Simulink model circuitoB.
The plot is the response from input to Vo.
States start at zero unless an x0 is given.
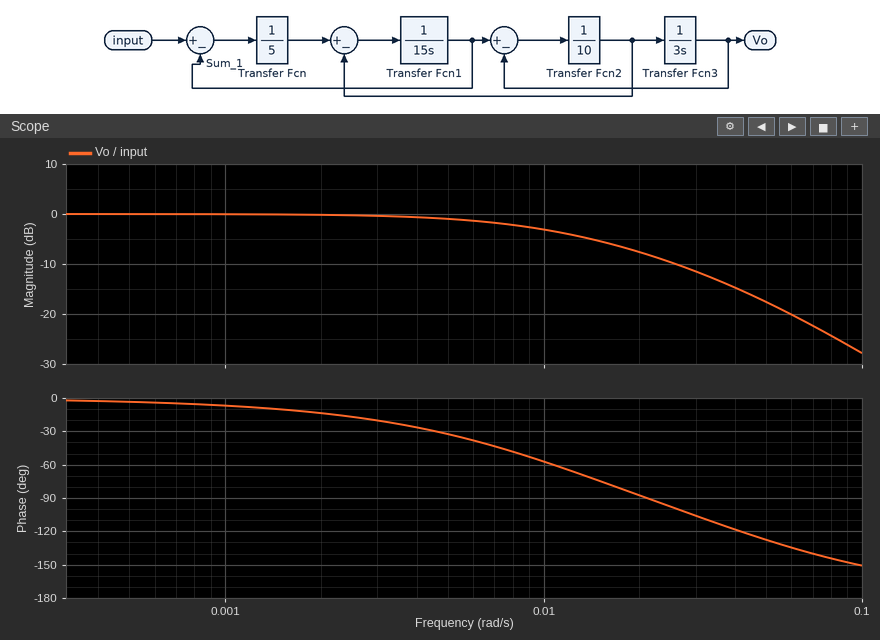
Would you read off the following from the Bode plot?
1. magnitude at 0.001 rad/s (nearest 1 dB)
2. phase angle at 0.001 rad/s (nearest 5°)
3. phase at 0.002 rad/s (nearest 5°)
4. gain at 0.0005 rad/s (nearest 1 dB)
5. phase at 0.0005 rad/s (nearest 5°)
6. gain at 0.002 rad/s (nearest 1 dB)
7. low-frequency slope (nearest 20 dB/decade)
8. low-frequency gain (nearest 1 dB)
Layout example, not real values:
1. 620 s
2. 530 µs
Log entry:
1. 0 dB
2. -5°
3. -15°
4. 0 dB
5. -5°
6. 0 dB
7. 0 dB/decade
8. 0 dB
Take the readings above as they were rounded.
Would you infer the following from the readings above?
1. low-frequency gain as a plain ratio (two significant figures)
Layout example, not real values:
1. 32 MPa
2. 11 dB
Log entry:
1. 1.0
